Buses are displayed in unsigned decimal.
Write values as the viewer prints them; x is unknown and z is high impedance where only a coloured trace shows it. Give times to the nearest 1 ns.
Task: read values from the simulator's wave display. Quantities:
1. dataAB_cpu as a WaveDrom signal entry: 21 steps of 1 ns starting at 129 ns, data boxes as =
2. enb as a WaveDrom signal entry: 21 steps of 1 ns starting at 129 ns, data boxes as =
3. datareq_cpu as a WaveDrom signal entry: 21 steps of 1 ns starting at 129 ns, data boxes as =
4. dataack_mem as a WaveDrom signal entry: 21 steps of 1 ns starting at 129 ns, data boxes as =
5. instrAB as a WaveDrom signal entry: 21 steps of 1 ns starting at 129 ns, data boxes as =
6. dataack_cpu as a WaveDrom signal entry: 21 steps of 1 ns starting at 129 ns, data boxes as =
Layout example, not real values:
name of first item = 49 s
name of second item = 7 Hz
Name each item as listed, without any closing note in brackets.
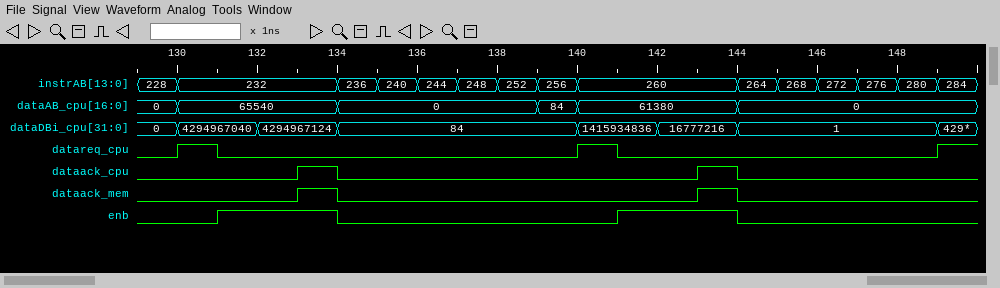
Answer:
dataAB_cpu as a WaveDrom signal entry: 21 steps of 1 ns starting at 129 ns, data boxes as = = {name: 'dataAB_cpu', wave: '==...=....==...=.....', data: '0 65540 0 84 61380 0'}
enb as a WaveDrom signal entry: 21 steps of 1 ns starting at 129 ns, data boxes as = = {name: 'enb', wave: '0.1..0......1..0.....'}
datareq_cpu as a WaveDrom signal entry: 21 steps of 1 ns starting at 129 ns, data boxes as = = {name: 'datareq_cpu', wave: '010........10.......1'}
dataack_mem as a WaveDrom signal entry: 21 steps of 1 ns starting at 129 ns, data boxes as = = {name: 'dataack_mem', wave: '0...10........10.....'}
instrAB as a WaveDrom signal entry: 21 steps of 1 ns starting at 129 ns, data boxes as = = {name: 'instrAB', wave: '==...=======...======', data: '228 232 236 240 244 248 252 256 260 264 268 272 276 280 284'}
dataack_cpu as a WaveDrom signal entry: 21 steps of 1 ns starting at 129 ns, data boxes as = = {name: 'dataack_cpu', wave: '0...10........10.....'}
